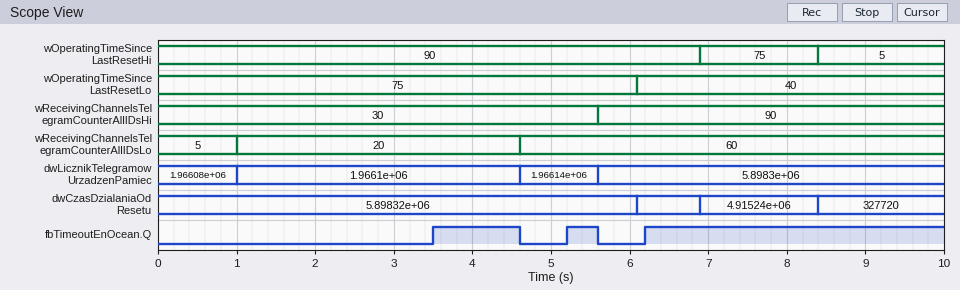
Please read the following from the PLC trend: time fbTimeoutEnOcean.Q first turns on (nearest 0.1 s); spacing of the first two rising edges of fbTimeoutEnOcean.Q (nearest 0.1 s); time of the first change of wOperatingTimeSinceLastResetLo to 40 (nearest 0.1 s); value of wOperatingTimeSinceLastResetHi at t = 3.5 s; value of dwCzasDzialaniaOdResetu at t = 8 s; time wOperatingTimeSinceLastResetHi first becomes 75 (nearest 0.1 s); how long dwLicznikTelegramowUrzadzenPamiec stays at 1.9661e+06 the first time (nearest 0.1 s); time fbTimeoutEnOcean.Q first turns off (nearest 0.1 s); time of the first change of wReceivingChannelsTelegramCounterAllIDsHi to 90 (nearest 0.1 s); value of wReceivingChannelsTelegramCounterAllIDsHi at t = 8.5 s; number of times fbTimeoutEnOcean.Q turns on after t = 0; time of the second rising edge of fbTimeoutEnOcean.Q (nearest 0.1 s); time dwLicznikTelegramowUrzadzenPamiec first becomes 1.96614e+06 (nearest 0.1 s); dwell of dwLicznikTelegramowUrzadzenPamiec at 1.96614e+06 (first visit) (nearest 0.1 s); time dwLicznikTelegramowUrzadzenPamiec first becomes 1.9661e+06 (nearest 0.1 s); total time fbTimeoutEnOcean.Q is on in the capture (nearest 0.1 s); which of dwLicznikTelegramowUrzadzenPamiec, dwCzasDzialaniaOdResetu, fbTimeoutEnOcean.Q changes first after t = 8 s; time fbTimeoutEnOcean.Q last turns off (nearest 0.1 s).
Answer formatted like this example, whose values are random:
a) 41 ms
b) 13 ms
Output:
a) 3.5 s
b) 1.7 s
c) 6.1 s
d) 90
e) 4.91524e+06
f) 6.9 s
g) 3.6 s
h) 4.6 s
i) 5.6 s
j) 90
k) 3
l) 5.2 s
m) 4.6 s
n) 1.0 s
o) 1.0 s
p) 5.3 s
q) dwCzasDzialaniaOdResetu
r) 5.6 s
